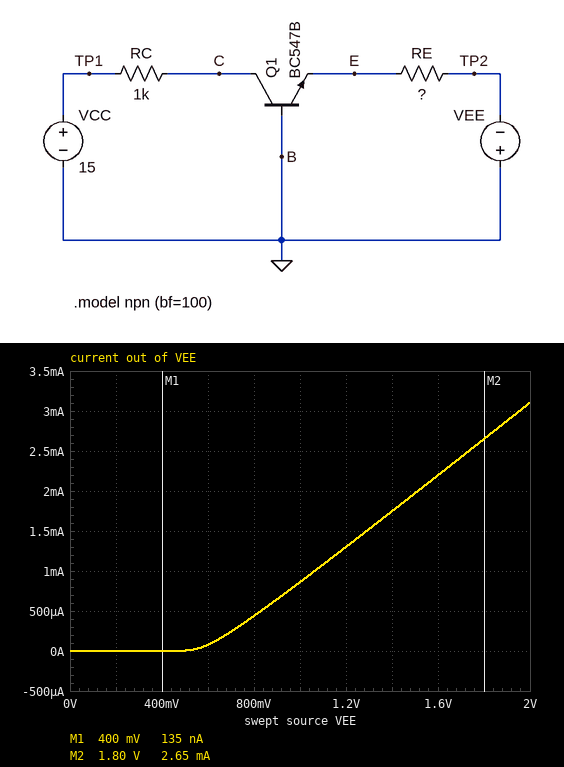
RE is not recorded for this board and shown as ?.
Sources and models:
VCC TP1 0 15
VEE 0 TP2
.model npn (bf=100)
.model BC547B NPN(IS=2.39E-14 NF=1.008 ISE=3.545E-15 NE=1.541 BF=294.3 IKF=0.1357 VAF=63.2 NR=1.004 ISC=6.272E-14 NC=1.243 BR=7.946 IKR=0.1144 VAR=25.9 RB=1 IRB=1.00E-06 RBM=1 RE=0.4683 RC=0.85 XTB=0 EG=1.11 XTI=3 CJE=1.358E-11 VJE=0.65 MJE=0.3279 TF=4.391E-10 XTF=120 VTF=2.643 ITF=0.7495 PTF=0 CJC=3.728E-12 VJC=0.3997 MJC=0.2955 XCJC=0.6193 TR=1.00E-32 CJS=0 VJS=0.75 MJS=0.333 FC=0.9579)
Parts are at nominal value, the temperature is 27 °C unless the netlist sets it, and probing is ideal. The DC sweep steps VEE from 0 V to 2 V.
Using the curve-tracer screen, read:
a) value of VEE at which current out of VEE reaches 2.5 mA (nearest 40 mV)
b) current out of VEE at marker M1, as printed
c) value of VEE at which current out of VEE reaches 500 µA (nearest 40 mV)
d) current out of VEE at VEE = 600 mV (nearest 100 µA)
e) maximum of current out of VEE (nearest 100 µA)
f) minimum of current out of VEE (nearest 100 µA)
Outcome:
1.72 V
135 nA
840 mV
100 µA
3.1 mA
0 A
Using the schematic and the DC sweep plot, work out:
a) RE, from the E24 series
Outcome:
430 Ω
